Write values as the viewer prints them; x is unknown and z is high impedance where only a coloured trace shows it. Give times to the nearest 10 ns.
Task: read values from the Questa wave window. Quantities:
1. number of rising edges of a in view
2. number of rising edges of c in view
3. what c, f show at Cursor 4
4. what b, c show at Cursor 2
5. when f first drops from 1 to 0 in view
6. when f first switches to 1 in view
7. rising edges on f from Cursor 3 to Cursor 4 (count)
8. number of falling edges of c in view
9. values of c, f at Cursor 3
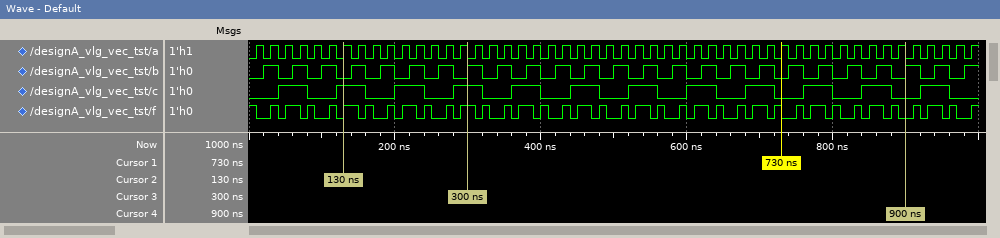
50
12
c=0, f=0
b=0, c=1
10 ns
30 ns
22
12
c=1, f=1
